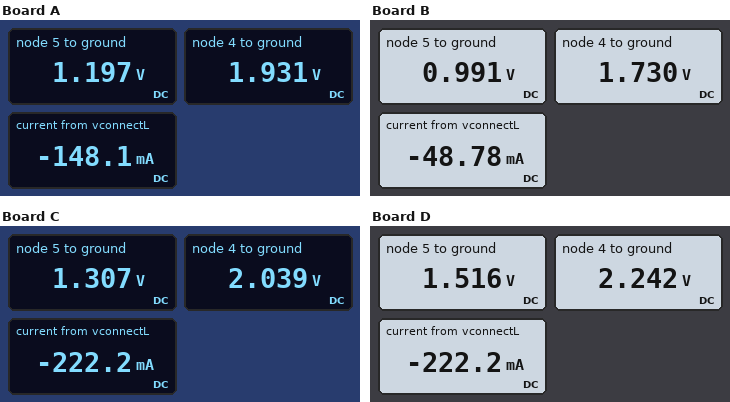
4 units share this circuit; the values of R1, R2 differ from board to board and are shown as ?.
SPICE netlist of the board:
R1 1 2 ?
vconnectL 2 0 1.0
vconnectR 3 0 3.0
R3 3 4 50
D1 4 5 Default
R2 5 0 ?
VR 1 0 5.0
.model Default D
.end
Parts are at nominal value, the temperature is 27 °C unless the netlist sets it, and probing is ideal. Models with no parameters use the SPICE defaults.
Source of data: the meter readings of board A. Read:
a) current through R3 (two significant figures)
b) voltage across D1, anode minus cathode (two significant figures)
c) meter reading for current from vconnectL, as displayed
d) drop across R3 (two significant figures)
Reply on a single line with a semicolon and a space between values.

21 mA; 730 mV; -148.1 mA; 1.1 V
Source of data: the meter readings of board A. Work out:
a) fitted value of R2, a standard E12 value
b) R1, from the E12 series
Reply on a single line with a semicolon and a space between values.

56 Ω; 27 Ω
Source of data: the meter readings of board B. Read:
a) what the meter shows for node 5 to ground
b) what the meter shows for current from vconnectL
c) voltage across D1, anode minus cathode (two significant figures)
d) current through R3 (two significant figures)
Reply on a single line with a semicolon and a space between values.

0.991 V; -48.78 mA; 740 mV; 25 mA
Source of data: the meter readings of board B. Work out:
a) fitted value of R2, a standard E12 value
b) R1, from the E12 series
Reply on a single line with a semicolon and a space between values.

39 Ω; 82 Ω
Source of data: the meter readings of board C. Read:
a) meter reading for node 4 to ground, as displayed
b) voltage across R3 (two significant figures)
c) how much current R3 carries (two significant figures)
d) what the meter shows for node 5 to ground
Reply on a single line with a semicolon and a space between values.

2.039 V; 960 mV; 19 mA; 1.307 V
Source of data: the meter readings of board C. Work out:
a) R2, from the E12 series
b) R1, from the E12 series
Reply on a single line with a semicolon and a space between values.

68 Ω; 18 Ω
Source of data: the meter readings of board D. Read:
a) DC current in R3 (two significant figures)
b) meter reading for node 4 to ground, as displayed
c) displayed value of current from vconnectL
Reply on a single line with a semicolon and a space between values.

15 mA; 2.242 V; -222.2 mA
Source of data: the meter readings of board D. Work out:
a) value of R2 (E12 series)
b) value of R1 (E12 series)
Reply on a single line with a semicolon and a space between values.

100 Ω; 18 Ω
